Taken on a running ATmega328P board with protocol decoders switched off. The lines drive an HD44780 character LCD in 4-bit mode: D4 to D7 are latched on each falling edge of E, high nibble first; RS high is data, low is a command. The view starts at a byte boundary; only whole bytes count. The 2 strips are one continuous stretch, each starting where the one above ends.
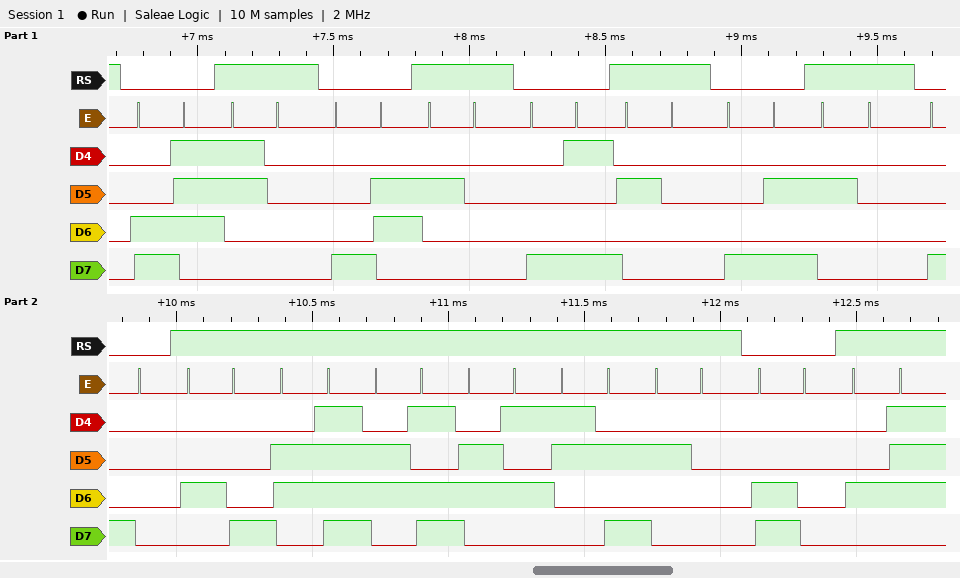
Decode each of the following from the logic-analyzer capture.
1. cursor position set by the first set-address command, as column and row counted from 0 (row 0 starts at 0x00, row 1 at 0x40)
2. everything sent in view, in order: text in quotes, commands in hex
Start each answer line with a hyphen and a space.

- column 7, row 1
- 0xC7 "0" 0x86 " " 0x89 " " 0x8A " " 0x80 "Home: " 0xC0 "G"
